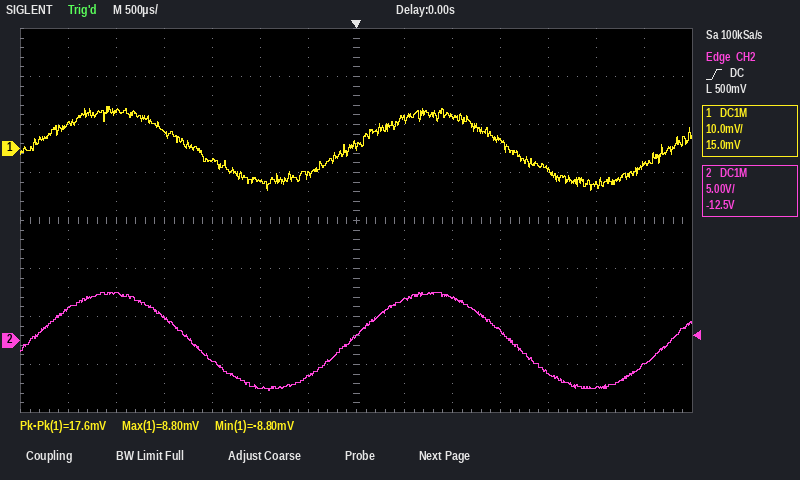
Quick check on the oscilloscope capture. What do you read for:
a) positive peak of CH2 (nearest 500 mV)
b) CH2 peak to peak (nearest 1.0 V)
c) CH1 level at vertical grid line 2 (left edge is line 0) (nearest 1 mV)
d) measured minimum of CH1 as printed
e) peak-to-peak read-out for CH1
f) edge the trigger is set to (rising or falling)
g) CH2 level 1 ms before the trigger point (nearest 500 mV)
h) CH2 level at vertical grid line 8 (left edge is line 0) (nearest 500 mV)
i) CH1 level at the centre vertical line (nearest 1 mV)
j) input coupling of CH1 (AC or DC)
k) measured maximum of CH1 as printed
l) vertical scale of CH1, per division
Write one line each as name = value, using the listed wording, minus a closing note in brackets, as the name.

positive peak of CH2 = 5.0 V
CH2 peak to peak = 10.0 V
CH1 level at vertical grid line 2 (left edge is line 0) = 8 mV
measured minimum of CH1 as printed = -8.80 mV
peak-to-peak read-out for CH1 = 17.6 mV
edge the trigger is set to = rising
CH2 level 1 ms before the trigger point = -5.0 V
CH2 level at vertical grid line 8 (left edge is line 0) = 4.5 V
CH1 level at the centre vertical line = 1 mV
input coupling of CH1 = DC
measured maximum of CH1 as printed = 8.80 mV
vertical scale of CH1, per division = 10 mV
